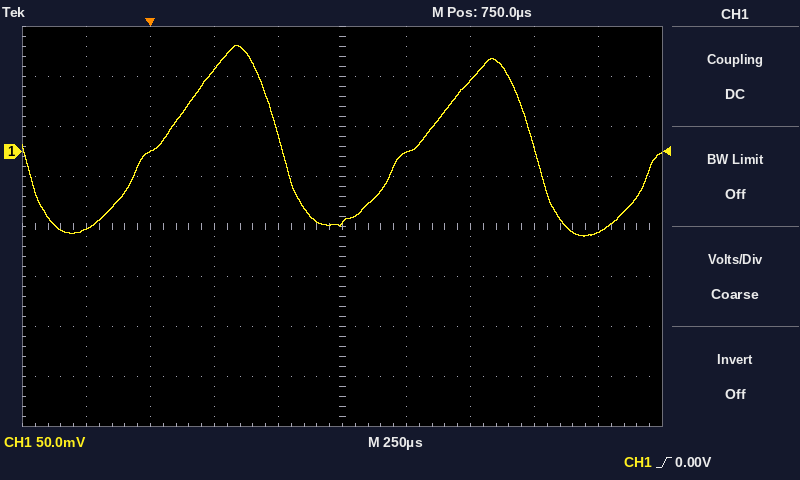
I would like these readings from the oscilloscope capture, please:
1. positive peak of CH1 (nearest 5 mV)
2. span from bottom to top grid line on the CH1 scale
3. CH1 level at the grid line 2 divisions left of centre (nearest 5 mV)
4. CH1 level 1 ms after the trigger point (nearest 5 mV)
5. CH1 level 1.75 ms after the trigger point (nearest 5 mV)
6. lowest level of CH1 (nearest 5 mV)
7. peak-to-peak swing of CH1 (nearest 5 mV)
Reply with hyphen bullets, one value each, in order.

- 105 mV
- 400 mV
- 80 mV
- 0 mV
- -80 mV
- -85 mV
- 190 mV
